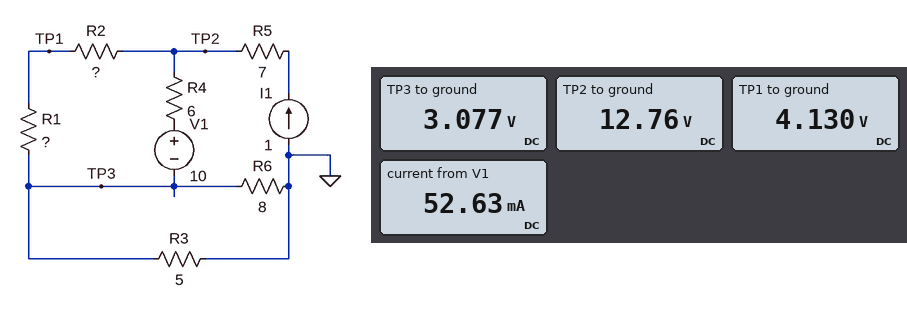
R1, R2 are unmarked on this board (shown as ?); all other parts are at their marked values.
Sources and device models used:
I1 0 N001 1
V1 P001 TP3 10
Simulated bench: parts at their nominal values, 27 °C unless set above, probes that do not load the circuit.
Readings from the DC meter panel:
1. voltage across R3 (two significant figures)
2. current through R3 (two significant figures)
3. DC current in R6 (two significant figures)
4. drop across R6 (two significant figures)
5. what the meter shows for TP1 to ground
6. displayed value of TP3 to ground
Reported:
3.1 V
620 mA
380 mA
3.1 V
4.130 V
3.077 V
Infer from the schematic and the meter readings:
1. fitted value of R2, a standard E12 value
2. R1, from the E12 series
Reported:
8.2 Ω
1 Ω
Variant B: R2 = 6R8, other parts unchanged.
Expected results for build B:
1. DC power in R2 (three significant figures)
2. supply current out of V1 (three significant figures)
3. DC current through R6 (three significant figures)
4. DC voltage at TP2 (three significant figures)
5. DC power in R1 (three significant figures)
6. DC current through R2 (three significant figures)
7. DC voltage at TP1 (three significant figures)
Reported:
9.14 W
159 mA
385 mA
12.1 V
1.34 W
1.16 A
4.24 V
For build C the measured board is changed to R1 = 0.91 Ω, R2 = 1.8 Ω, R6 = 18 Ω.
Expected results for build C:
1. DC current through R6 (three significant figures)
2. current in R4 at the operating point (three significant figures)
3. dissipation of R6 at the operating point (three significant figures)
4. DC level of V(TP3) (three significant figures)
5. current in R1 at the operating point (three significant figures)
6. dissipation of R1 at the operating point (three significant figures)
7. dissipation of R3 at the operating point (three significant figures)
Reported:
217 mA
837 mA
851 mW
3.91 V
1.84 A
3.07 W
3.06 W
